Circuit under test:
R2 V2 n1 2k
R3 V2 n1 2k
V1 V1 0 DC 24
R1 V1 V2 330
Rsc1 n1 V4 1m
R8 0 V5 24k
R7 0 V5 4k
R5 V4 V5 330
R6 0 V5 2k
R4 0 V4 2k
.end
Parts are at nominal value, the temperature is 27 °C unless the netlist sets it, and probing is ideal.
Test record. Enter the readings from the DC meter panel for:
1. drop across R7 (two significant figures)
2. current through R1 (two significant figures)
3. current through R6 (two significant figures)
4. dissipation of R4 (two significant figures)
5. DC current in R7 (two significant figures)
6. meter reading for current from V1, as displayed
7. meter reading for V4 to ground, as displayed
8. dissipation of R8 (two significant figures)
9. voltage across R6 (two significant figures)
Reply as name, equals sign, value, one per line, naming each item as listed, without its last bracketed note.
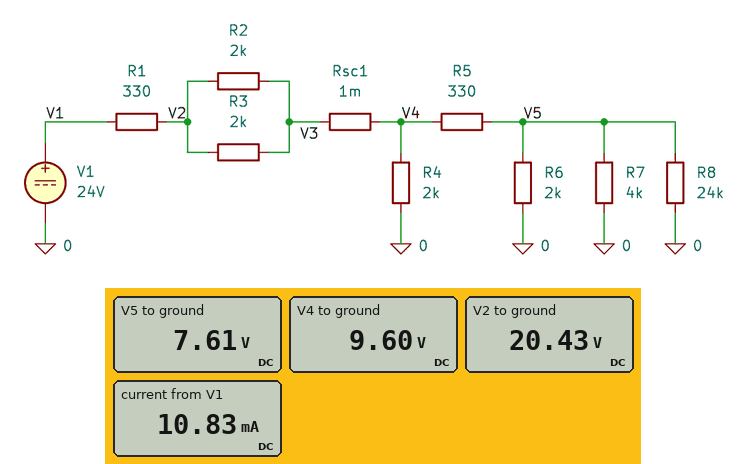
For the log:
drop across R7 = 7.6 V
current through R1 = 11 mA
current through R6 = 3.8 mA
dissipation of R4 = 46 mW
DC current in R7 = 1.9 mA
meter reading for current from V1, as displayed = 10.83 mA
meter reading for V4 to ground, as displayed = 9.60 V
dissipation of R8 = 2.4 mW
voltage across R6 = 7.6 V
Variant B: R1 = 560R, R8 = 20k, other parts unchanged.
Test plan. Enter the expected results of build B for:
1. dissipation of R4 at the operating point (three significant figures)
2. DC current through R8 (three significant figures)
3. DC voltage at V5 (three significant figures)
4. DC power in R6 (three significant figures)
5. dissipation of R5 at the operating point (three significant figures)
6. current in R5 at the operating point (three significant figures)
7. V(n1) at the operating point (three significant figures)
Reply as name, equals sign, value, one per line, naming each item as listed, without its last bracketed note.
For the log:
dissipation of R4 at the operating point = 37.6 mW
DC current through R8 = 343 µA
DC voltage at V5 = 6.86 V
DC power in R6 = 23.5 mW
dissipation of R5 at the operating point = 9.94 mW
current in R5 at the operating point = 5.49 mA
V(n1) at the operating point = 8.67 V
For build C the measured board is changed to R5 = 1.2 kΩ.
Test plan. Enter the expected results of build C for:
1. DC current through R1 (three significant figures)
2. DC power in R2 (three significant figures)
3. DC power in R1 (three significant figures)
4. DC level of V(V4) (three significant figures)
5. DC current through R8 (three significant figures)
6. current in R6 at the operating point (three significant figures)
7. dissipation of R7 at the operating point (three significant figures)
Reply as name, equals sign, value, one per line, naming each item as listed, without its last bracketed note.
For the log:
DC current through R1 = 9.86 mA
DC power in R2 = 48.6 mW
DC power in R1 = 32.1 mW
DC level of V(V4) = 10.9 V
DC current through R8 = 233 µA
current in R6 at the operating point = 2.79 mA
dissipation of R7 at the operating point = 7.79 mW
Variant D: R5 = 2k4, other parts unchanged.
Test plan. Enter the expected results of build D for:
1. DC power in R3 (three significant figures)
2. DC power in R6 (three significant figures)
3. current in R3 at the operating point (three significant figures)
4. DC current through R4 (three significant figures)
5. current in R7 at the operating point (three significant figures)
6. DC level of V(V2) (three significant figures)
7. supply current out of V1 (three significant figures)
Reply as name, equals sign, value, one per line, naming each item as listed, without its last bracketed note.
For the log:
DC power in R3 = 41.8 mW
DC power in R6 = 8.33 mW
current in R3 at the operating point = 4.57 mA
DC current through R4 = 5.92 mA
current in R7 at the operating point = 1.02 mA
DC level of V(V2) = 21.0 V
supply current out of V1 = 9.15 mA
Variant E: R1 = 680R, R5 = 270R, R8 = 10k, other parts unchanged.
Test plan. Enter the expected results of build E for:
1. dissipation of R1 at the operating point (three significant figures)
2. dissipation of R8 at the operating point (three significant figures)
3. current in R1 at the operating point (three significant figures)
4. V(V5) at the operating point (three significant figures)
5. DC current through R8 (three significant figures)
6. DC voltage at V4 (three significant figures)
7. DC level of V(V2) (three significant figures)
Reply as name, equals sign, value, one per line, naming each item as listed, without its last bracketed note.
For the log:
dissipation of R1 at the operating point = 61.7 mW
dissipation of R8 at the operating point = 4.23 mW
current in R1 at the operating point = 9.53 mA
V(V5) at the operating point = 6.50 V
DC current through R8 = 650 µA
DC voltage at V4 = 8.00 V
DC level of V(V2) = 17.5 V
